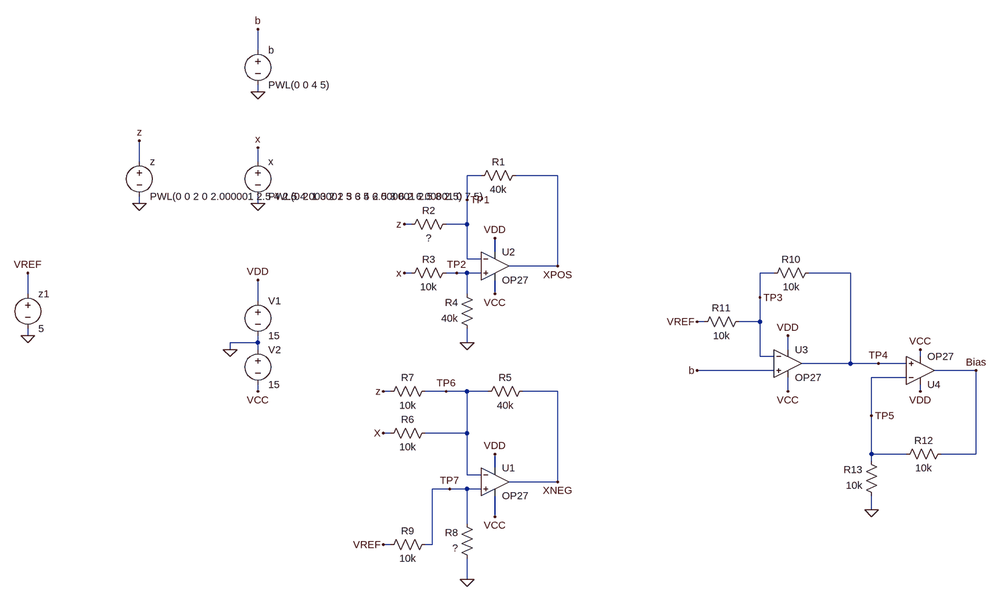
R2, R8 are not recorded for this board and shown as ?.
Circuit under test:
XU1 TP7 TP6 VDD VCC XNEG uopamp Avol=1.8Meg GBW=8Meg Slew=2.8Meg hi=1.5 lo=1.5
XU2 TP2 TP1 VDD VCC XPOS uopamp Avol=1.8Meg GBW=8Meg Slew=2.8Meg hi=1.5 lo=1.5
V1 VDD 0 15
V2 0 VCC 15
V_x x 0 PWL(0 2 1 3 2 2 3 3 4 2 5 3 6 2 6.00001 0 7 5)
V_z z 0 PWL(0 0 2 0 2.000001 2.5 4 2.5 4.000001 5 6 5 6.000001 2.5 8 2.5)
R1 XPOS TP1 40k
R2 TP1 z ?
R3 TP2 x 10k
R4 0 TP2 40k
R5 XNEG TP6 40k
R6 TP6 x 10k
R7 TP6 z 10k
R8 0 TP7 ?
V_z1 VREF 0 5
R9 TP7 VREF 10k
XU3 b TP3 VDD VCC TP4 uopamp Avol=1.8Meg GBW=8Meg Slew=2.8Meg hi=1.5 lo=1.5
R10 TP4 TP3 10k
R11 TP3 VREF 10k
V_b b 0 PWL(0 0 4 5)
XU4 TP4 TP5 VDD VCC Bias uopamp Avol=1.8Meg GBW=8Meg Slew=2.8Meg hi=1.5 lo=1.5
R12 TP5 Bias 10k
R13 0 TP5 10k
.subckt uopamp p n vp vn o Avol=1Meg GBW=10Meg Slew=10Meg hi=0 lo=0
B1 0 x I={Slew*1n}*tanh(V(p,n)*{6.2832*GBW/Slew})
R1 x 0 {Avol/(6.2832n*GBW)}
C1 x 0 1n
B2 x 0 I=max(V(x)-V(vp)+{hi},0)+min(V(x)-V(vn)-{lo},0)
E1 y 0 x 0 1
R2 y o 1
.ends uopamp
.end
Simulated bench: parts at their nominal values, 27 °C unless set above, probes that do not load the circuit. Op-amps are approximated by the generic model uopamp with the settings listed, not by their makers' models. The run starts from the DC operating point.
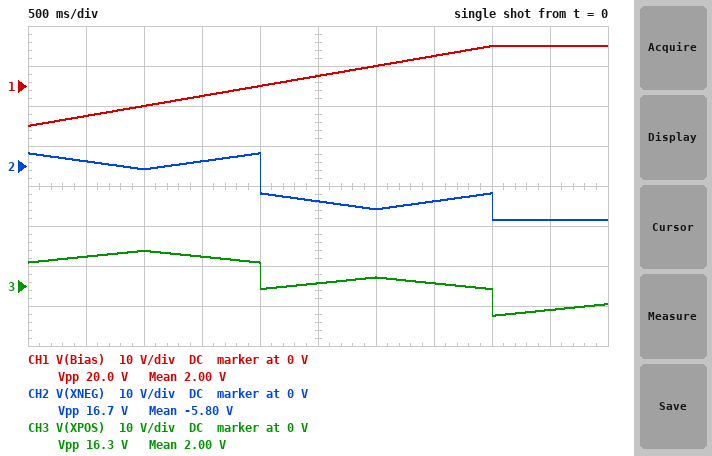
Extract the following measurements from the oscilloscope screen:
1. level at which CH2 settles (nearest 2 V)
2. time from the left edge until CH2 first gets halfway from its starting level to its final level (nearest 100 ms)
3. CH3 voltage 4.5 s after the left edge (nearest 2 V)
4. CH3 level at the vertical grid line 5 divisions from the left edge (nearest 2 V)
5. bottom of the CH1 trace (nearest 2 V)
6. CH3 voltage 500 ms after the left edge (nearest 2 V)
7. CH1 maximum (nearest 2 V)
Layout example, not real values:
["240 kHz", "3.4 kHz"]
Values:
["-14 V", "2.0 s", "-6 V", "0 V", "-10 V", "8 V", "10 V"]
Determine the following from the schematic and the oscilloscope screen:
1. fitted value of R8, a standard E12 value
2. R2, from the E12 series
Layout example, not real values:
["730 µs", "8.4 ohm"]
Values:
["3.3 kΩ", "15 kΩ"]
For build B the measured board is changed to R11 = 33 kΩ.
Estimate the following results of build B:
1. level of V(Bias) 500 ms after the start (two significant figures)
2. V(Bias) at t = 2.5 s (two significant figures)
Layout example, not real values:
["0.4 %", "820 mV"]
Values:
["-1.4 V", "5.1 V"]
